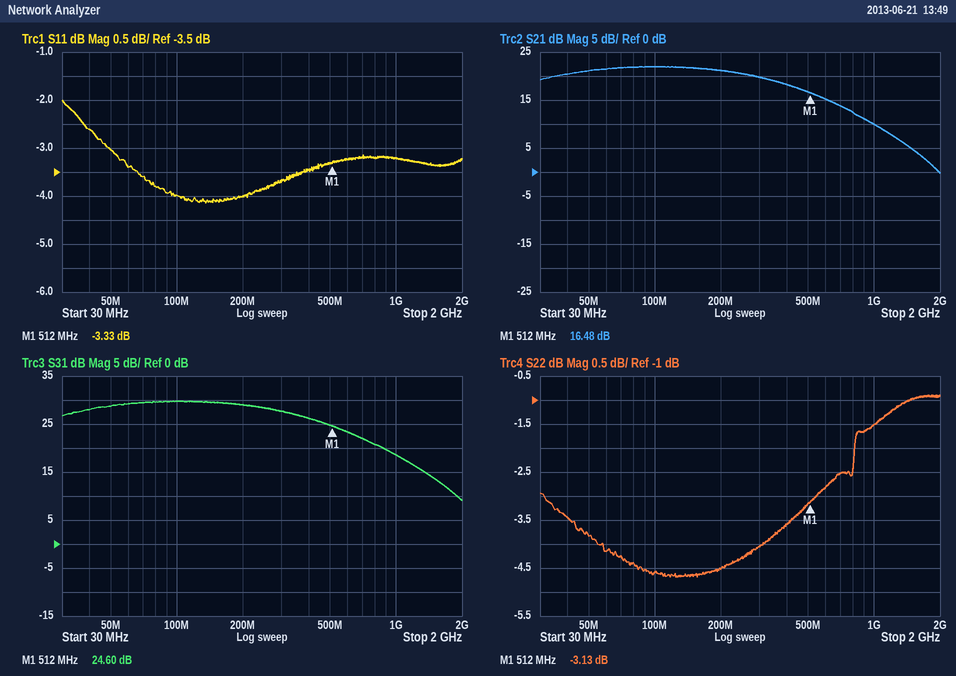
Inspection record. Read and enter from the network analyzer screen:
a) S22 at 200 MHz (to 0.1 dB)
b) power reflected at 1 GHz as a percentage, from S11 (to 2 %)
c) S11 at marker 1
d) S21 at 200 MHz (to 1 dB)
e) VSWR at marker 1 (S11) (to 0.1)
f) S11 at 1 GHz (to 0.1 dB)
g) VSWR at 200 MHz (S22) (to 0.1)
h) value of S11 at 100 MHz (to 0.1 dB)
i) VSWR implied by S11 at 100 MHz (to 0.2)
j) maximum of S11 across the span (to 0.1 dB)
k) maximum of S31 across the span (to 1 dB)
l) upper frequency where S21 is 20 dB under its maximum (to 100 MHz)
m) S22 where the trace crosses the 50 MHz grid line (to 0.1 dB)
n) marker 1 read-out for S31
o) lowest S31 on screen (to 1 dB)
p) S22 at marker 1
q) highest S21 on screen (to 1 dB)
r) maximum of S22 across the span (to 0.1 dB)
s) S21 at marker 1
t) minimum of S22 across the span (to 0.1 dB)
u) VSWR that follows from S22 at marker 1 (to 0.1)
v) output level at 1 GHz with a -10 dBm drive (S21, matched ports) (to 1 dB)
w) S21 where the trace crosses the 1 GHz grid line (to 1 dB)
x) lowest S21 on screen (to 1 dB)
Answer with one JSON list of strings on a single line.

["-4.5 dB", "48 %", "-3.33 dB", "21 dB", "5.3", "-3.2 dB", "3.9", "-4.0 dB", "4.4", "-2.0 dB", "30 dB", "1.8 GHz", "-3.8 dB", "24.60 dB", "9 dB", "-3.13 dB", "22 dB", "-0.9 dB", "16.48 dB", "-4.7 dB", "5.6", "0 dBm", "10 dB", "0 dB"]
